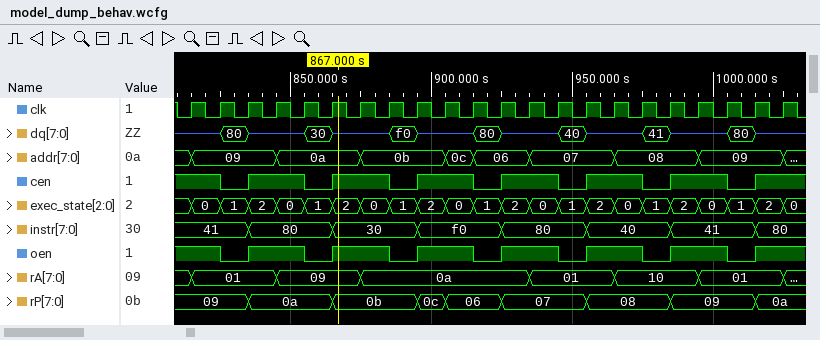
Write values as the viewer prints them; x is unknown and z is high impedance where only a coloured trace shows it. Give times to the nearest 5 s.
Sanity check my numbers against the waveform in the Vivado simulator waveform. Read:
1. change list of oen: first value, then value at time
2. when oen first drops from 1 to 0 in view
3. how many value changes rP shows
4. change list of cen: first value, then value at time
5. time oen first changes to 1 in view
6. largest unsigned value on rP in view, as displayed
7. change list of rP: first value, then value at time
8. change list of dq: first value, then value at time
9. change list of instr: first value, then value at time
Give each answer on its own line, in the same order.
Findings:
1, 0 at 825 s, 1 at 835 s, 0 at 855 s, 1 at 865 s, 0 at 885 s, 1 at 895 s, 0 at 915 s, 1 at 925 s, 0 at 945 s, 1 at 955 s, 0 at 975 s, 1 at 985 s, 0 at 1005 s, 1 at 1015 s
825 s
8
1, 0 at 825 s, 1 at 835 s, 0 at 855 s, 1 at 865 s, 0 at 885 s, 1 at 895 s, 0 at 915 s, 1 at 925 s, 0 at 945 s, 1 at 955 s, 0 at 975 s, 1 at 985 s, 0 at 1005 s, 1 at 1015 s
835 s
0c
09, 0a at 835 s, 0b at 865 s, 0c at 895 s, 06 at 905 s, 07 at 925 s, 08 at 955 s, 09 at 985 s, 0a at 1015 s
z, 80 at 825 s, z at 835 s, 30 at 855 s, z at 865 s, f0 at 885 s, z at 895 s, 80 at 915 s, z at 925 s, 40 at 945 s, z at 955 s, 41 at 975 s, z at 985 s, 80 at 1005 s, z at 1015 s
41, 80 at 835 s, 30 at 865 s, f0 at 895 s, 80 at 925 s, 40 at 955 s, 41 at 985 s, 80 at 1015 s
